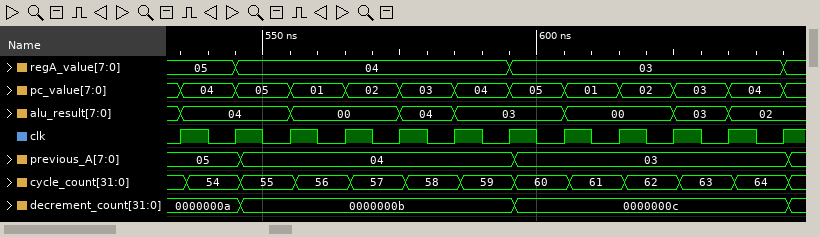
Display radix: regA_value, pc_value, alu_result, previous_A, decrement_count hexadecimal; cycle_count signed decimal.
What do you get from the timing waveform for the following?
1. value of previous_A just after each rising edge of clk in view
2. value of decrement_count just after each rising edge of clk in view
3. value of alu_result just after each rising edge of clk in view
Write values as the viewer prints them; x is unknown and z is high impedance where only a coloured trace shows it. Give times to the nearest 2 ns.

05, 05, 04, 04, 04, 04, 04, 03, 03, 03, 03, 03
0000000a, 0000000a, 0000000b, 0000000b, 0000000b, 0000000b, 0000000b, 0000000c, 0000000c, 0000000c, 0000000c, 0000000c
04, 04, 00, 00, 04, 03, 03, 00, 00, 03, 02, 02
